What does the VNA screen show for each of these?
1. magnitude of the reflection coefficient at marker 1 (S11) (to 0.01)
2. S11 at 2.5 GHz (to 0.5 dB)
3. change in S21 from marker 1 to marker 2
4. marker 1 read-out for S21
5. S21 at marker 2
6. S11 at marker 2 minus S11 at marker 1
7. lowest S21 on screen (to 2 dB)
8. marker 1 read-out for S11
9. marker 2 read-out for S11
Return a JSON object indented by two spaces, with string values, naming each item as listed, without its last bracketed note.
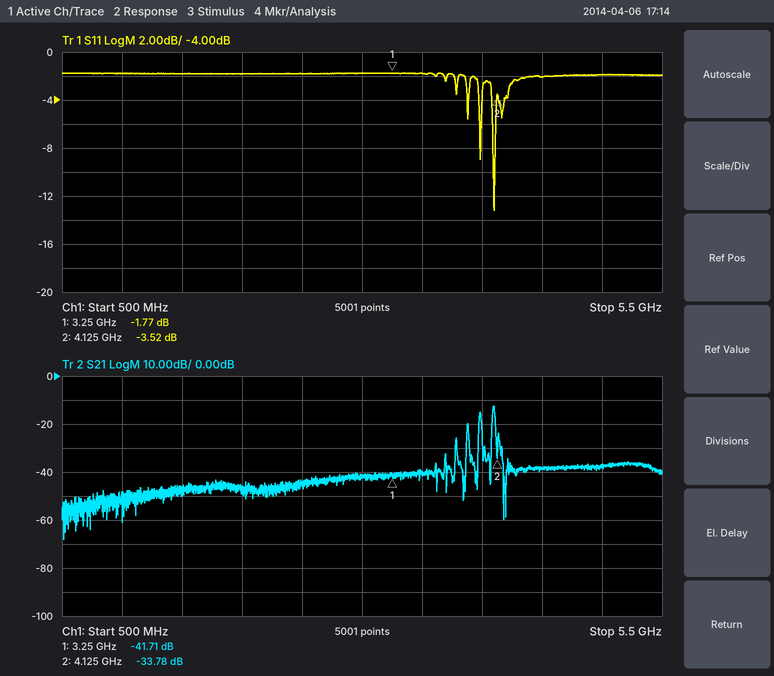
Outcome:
{
  "magnitude of the reflection coefficient at marker 1 (S11)": "0.82",
  "S11 at 2.5 GHz": "-2.0 dB",
  "change in S21 from marker 1 to marker 2": "7.93 dB",
  "marker 1 read-out for S21": "-41.71 dB",
  "S21 at marker 2": "-33.78 dB",
  "S11 at marker 2 minus S11 at marker 1": "-1.75 dB",
  "lowest S21 on screen": "-68 dB",
  "marker 1 read-out for S11": "-1.77 dB",
  "marker 2 read-out for S11": "-3.52 dB"
}
